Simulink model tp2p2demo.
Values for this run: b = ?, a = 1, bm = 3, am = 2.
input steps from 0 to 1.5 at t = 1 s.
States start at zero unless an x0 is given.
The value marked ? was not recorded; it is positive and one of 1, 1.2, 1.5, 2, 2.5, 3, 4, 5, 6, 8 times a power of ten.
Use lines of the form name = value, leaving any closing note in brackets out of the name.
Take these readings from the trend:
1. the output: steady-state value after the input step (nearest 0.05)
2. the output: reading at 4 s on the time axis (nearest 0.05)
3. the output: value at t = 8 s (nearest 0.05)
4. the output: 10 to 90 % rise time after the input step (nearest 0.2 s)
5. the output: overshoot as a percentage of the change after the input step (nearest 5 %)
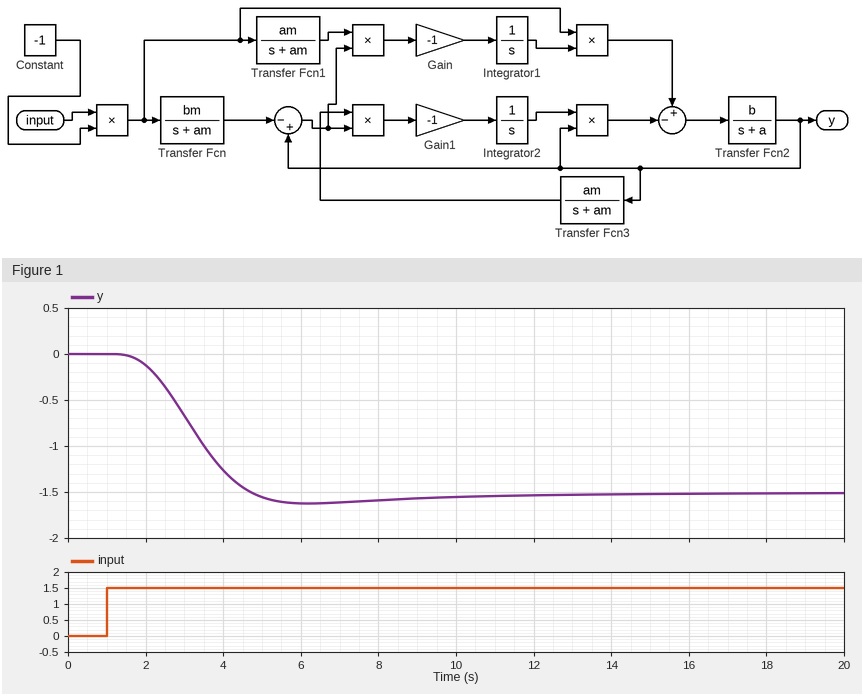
the output: steady-state value after the input step = -1.50
the output: reading at 4 s on the time axis = -1.25
the output: value at t = 8 s = -1.60
the output: 10 to 90 % rise time after the input step = 2.2 s
the output: overshoot as a percentage of the change after the input step = 10 %
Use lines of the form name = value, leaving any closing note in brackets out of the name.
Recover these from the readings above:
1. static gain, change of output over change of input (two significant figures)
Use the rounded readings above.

static gain, change of output over change of input = -1.0
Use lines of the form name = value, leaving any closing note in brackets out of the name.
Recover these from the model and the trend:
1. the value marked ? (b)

the value marked ? = 0.25
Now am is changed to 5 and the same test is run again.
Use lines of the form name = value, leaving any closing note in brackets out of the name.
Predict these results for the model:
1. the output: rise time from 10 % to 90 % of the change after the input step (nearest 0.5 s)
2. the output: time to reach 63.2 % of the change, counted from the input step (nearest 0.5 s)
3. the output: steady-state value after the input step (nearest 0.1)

the output: rise time from 10 % to 90 % of the change after the input step = 3.0 s
the output: time to reach 63.2 % of the change, counted from the input step = 2.5 s
the output: steady-state value after the input step = -0.9
